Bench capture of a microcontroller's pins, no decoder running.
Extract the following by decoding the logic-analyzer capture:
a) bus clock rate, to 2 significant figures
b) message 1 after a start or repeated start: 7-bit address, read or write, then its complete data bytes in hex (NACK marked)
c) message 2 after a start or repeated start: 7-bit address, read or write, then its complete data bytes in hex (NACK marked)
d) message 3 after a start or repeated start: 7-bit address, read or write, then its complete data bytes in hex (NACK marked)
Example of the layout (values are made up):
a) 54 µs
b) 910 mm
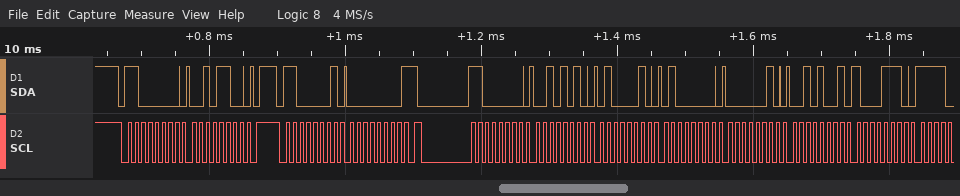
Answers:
a) 100 kHz
b) 0x60 write: 2C
c) 0x60 read: 00 NACK
d) 0x60 write: 2A 42 40 02 29 8E
